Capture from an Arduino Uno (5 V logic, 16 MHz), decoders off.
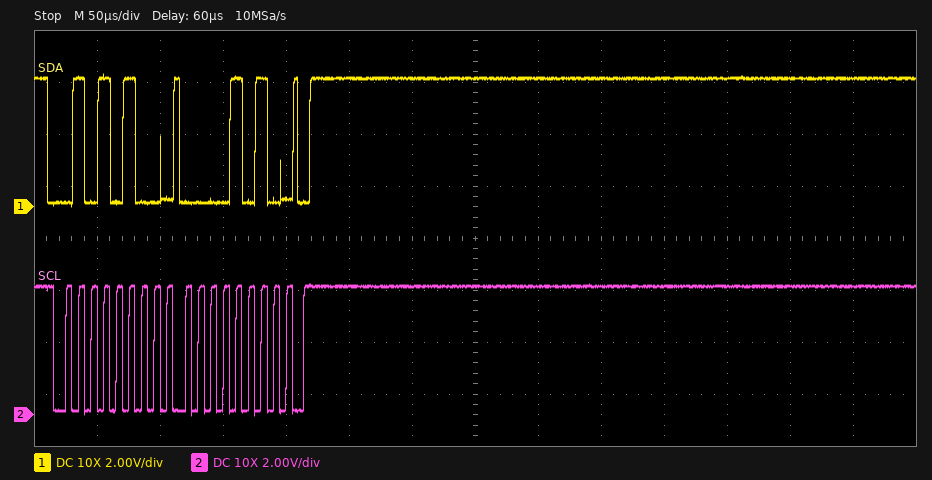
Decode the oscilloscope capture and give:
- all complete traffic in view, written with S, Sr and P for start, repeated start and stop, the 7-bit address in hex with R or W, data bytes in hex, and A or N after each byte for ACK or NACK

S 2AW A 0A A P
